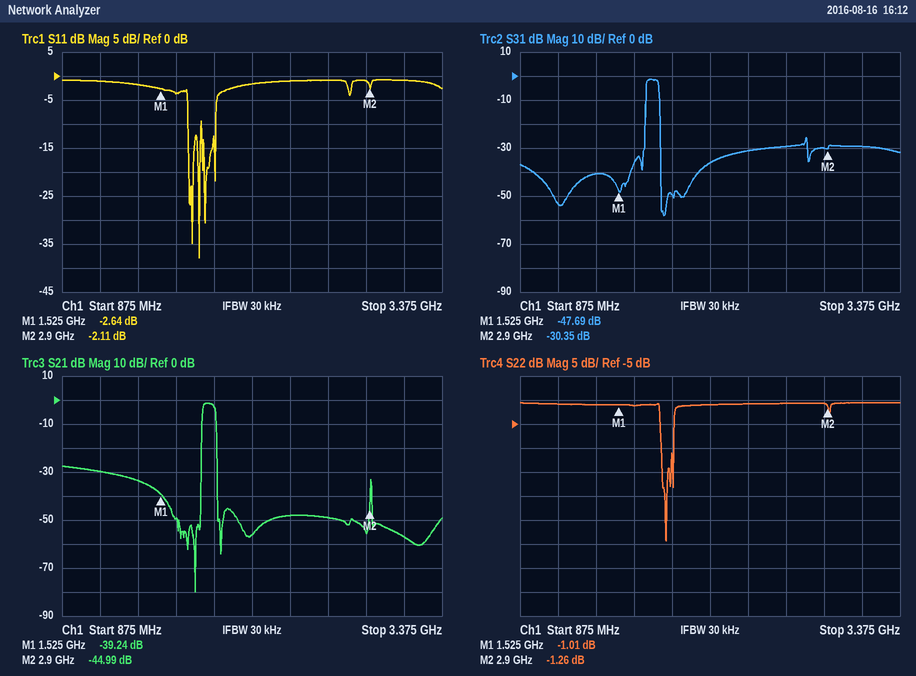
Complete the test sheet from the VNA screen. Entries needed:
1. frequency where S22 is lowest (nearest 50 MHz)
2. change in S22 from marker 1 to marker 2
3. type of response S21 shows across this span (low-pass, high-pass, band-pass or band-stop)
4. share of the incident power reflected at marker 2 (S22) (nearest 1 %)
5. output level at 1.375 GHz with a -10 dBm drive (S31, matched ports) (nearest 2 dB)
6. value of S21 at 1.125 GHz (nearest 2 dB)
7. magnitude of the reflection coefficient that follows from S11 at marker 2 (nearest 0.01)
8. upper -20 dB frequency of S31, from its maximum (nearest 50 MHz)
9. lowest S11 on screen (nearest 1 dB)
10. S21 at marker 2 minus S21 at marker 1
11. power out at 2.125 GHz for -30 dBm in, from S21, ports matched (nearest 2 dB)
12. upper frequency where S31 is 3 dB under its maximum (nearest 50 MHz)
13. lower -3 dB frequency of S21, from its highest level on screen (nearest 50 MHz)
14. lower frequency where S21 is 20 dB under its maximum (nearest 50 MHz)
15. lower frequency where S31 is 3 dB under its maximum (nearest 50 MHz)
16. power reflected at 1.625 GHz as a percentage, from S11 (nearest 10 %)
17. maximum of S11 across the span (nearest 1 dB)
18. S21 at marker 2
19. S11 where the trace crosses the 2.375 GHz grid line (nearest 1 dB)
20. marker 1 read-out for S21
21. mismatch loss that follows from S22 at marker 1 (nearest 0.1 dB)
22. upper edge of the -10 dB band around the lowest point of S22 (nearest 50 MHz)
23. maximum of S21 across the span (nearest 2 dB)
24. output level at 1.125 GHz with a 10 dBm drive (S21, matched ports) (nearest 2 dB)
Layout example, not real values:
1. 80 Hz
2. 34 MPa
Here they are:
1. 1.85 GHz
2. -0.25 dB
3. band-pass
4. 75 %
5. -50 dBm
6. -30 dB
7. 0.78
8. 1.80 GHz
9. -38 dB
10. -5.75 dB
11. -86 dBm
12. 1.80 GHz
13. 1.80 GHz
14. 1.80 GHz
15. 1.70 GHz
16. 40 %
17. -1 dB
18. -44.99 dB
19. -1 dB
20. -39.24 dB
21. 6.8 dB
22. 1.90 GHz
23. -2 dB
24. -20 dBm
